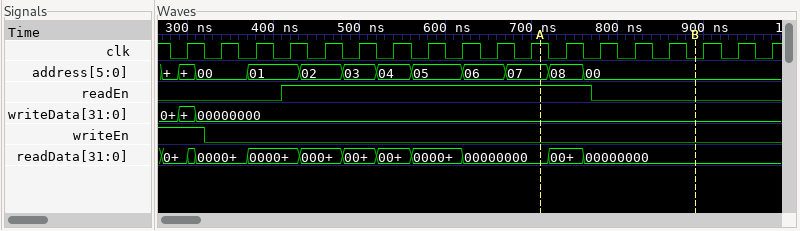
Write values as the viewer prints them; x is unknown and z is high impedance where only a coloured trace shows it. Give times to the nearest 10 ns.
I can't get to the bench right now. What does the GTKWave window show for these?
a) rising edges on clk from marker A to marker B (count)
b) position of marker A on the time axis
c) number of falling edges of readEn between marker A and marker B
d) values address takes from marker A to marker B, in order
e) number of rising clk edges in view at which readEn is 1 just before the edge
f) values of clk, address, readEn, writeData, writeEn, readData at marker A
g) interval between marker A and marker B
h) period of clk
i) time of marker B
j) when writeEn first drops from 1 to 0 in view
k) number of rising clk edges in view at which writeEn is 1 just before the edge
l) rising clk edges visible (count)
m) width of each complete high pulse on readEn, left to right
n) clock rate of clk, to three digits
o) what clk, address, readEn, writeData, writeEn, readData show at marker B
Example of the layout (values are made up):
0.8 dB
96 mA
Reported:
4
710 ns
1
07, 08, 00
9
clk=1, address=07, readEn=1, writeData=00000000, writeEn=0, readData=00000000
180 ns
40 ns
890 ns
320 ns
1
18
360 ns
25.0 MHz
clk=0, address=00, readEn=0, writeData=00000000, writeEn=0, readData=00000000
